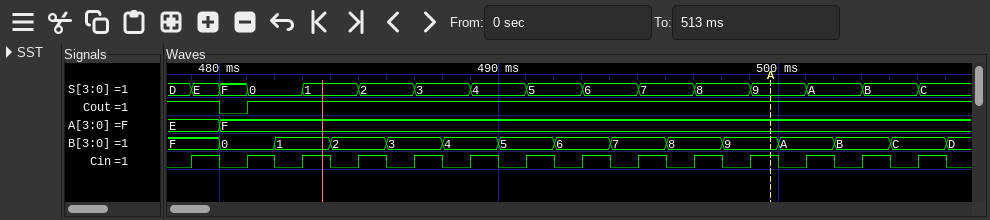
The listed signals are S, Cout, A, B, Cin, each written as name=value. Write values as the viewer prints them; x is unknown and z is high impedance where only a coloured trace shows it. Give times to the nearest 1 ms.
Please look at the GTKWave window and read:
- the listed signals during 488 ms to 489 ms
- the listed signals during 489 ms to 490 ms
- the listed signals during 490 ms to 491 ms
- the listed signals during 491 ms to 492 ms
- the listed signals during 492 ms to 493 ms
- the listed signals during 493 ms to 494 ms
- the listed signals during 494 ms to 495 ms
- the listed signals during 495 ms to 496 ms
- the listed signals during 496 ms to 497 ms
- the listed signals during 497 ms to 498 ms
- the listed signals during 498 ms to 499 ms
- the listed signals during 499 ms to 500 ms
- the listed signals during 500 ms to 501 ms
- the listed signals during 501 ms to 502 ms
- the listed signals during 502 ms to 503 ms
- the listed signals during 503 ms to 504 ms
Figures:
S=3, Cout=1, A=F, B=4, Cin=0
S=4, Cout=1, A=F, B=4, Cin=1
S=4, Cout=1, A=F, B=5, Cin=0
S=5, Cout=1, A=F, B=5, Cin=1
S=5, Cout=1, A=F, B=6, Cin=0
S=6, Cout=1, A=F, B=6, Cin=1
S=6, Cout=1, A=F, B=7, Cin=0
S=7, Cout=1, A=F, B=7, Cin=1
S=7, Cout=1, A=F, B=8, Cin=0
S=8, Cout=1, A=F, B=8, Cin=1
S=8, Cout=1, A=F, B=9, Cin=0
S=9, Cout=1, A=F, B=9, Cin=1
S=9, Cout=1, A=F, B=A, Cin=0
S=A, Cout=1, A=F, B=A, Cin=1
S=A, Cout=1, A=F, B=B, Cin=0
S=B, Cout=1, A=F, B=B, Cin=1
